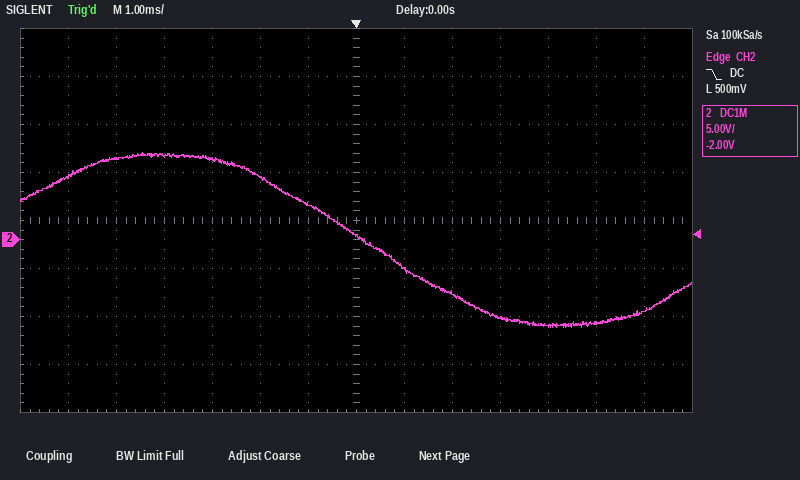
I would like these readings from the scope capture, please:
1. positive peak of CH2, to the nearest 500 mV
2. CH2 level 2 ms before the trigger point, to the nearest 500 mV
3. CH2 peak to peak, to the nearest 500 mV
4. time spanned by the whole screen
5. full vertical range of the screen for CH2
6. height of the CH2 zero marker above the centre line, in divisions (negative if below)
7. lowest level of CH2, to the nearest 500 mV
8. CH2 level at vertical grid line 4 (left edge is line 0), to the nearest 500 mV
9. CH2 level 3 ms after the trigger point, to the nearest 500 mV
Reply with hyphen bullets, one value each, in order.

- 9.0 V
- 6.5 V
- 18.0 V
- 14 ms
- 40 V
- -0.4 div
- -9.0 V
- 8.5 V
- -8.0 V
